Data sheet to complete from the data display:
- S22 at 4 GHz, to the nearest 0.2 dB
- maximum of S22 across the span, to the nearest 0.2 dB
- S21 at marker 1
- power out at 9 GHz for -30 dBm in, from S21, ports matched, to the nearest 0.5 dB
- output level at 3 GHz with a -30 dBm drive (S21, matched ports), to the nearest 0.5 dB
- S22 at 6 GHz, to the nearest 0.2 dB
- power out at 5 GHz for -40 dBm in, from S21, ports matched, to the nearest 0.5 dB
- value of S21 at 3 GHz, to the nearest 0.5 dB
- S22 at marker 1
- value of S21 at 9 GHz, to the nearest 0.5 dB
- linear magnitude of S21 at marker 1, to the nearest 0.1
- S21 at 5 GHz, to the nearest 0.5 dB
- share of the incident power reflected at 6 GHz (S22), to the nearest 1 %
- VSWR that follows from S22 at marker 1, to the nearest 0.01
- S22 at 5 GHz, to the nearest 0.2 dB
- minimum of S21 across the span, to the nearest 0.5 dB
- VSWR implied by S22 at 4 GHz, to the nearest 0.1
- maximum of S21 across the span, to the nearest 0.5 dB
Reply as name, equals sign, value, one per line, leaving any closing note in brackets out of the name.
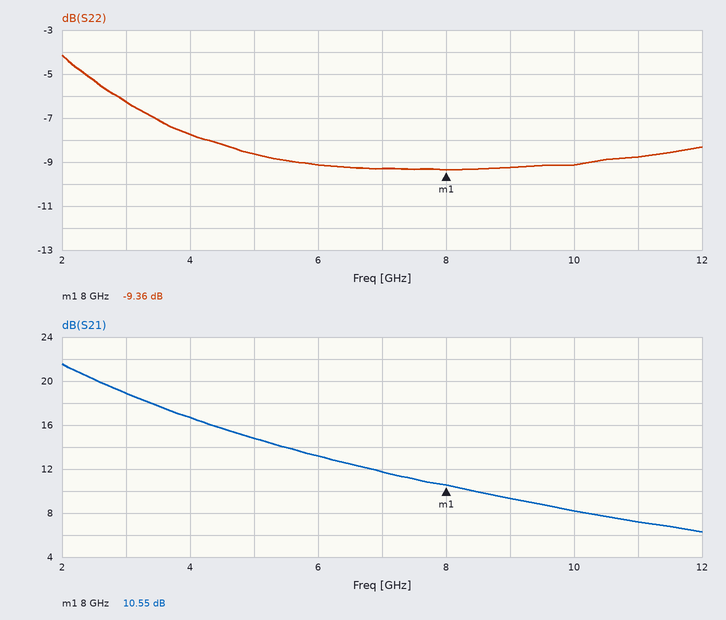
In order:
S22 at 4 GHz, to the nearest 0.2 dB = -7.8 dB
maximum of S22 across the span, to the nearest 0.2 dB = -4.2 dB
S21 at marker 1 = 10.55 dB
power out at 9 GHz for -30 dBm in, from S21, ports matched, to the nearest 0.5 dB = -20.5 dBm
output level at 3 GHz with a -30 dBm drive (S21, matched ports), to the nearest 0.5 dB = -11.0 dBm
S22 at 6 GHz, to the nearest 0.2 dB = -9.2 dB
power out at 5 GHz for -40 dBm in, from S21, ports matched, to the nearest 0.5 dB = -25.0 dBm
value of S21 at 3 GHz, to the nearest 0.5 dB = 19.0 dB
S22 at marker 1 = -9.36 dB
value of S21 at 9 GHz, to the nearest 0.5 dB = 9.5 dB
linear magnitude of S21 at marker 1, to the nearest 0.1 = 3.4
S21 at 5 GHz, to the nearest 0.5 dB = 15.0 dB
share of the incident power reflected at 6 GHz (S22), to the nearest 1 % = 12 %
VSWR that follows from S22 at marker 1, to the nearest 0.01 = 2.03
S22 at 5 GHz, to the nearest 0.2 dB = -8.6 dB
minimum of S21 across the span, to the nearest 0.5 dB = 6.5 dB
VSWR implied by S22 at 4 GHz, to the nearest 0.1 = 2.4
maximum of S21 across the span, to the nearest 0.5 dB = 21.5 dB
